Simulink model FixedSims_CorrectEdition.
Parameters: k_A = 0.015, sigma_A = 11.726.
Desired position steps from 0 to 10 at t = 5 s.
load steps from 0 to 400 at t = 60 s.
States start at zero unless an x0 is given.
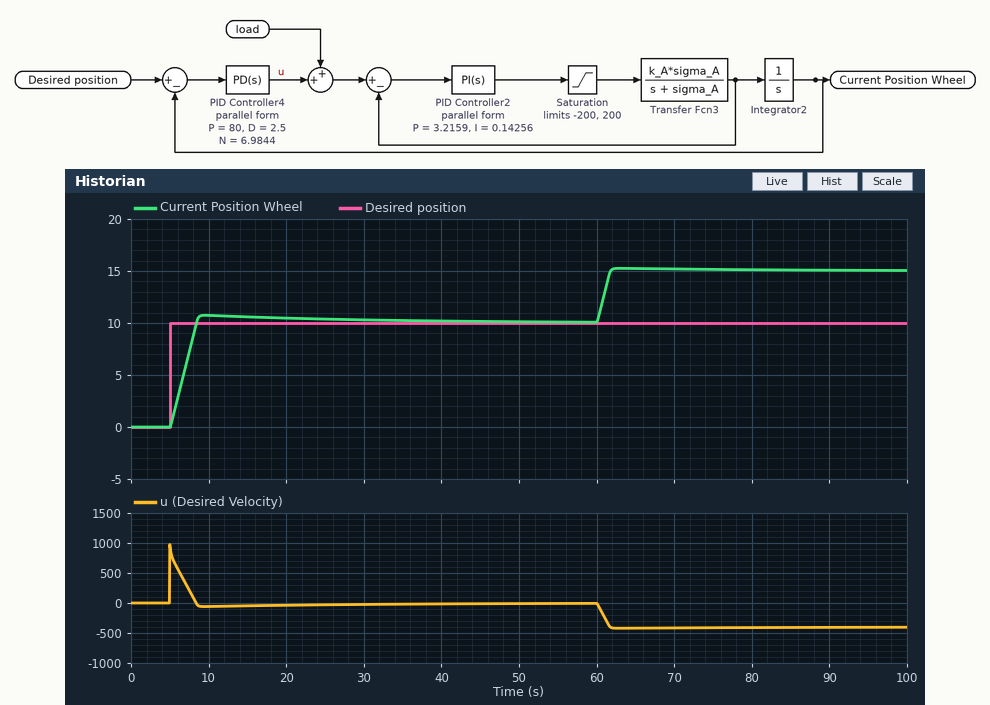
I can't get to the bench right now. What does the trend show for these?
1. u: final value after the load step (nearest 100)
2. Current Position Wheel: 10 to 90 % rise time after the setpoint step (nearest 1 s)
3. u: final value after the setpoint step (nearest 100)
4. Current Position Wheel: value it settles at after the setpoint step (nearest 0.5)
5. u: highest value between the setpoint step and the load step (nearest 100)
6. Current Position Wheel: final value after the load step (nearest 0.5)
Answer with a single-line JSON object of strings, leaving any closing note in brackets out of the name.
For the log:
{"u: final value after the load step": "-400", "Current Position Wheel: 10 to 90 % rise time after the setpoint step": "3 s", "u: final value after the setpoint step": "0", "Current Position Wheel: value it settles at after the setpoint step": "10.0", "u: highest value between the setpoint step and the load step": "1000", "Current Position Wheel: final value after the load step": "15.0"}
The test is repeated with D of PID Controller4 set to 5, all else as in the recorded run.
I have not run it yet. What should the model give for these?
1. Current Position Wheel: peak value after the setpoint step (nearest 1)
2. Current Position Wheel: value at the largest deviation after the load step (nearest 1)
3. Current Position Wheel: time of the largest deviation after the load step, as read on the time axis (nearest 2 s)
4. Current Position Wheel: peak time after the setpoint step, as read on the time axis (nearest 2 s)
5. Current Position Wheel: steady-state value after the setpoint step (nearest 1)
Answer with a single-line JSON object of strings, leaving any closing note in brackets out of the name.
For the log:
{"Current Position Wheel: peak value after the setpoint step": "11", "Current Position Wheel: value at the largest deviation after the load step": "15", "Current Position Wheel: time of the largest deviation after the load step, as read on the time axis": "64 s", "Current Position Wheel: peak time after the setpoint step, as read on the time axis": "10 s", "Current Position Wheel: steady-state value after the setpoint step": "10"}
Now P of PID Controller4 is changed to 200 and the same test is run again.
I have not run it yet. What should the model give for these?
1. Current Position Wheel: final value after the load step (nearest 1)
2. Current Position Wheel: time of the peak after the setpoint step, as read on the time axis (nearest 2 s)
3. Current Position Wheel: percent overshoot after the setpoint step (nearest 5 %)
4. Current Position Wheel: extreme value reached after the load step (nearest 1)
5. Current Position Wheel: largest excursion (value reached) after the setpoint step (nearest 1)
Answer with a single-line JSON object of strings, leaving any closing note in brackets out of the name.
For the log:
{"Current Position Wheel: final value after the load step": "12", "Current Position Wheel: time of the peak after the setpoint step, as read on the time axis": "8 s", "Current Position Wheel: percent overshoot after the setpoint step": "10 %", "Current Position Wheel: extreme value reached after the load step": "12", "Current Position Wheel: largest excursion (value reached) after the setpoint step": "11"}
